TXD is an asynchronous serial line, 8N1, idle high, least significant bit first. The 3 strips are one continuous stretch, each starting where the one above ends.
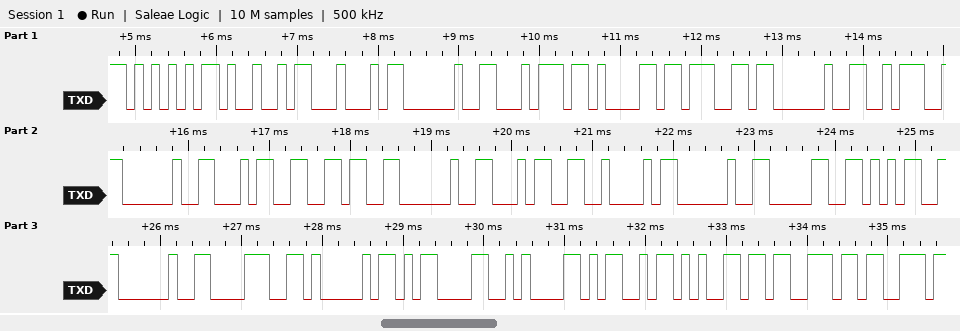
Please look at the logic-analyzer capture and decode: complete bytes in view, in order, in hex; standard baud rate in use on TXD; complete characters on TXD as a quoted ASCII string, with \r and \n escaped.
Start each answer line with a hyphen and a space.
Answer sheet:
- 55 49 44 20 74 61 67 20 3A 20 34 36 20 34 42 20 30 35 20 38 41 0D 0A 4D 65 73 73
- 9600 baud
- "UID tag : 46 4B 05 8A\r\nMess"
